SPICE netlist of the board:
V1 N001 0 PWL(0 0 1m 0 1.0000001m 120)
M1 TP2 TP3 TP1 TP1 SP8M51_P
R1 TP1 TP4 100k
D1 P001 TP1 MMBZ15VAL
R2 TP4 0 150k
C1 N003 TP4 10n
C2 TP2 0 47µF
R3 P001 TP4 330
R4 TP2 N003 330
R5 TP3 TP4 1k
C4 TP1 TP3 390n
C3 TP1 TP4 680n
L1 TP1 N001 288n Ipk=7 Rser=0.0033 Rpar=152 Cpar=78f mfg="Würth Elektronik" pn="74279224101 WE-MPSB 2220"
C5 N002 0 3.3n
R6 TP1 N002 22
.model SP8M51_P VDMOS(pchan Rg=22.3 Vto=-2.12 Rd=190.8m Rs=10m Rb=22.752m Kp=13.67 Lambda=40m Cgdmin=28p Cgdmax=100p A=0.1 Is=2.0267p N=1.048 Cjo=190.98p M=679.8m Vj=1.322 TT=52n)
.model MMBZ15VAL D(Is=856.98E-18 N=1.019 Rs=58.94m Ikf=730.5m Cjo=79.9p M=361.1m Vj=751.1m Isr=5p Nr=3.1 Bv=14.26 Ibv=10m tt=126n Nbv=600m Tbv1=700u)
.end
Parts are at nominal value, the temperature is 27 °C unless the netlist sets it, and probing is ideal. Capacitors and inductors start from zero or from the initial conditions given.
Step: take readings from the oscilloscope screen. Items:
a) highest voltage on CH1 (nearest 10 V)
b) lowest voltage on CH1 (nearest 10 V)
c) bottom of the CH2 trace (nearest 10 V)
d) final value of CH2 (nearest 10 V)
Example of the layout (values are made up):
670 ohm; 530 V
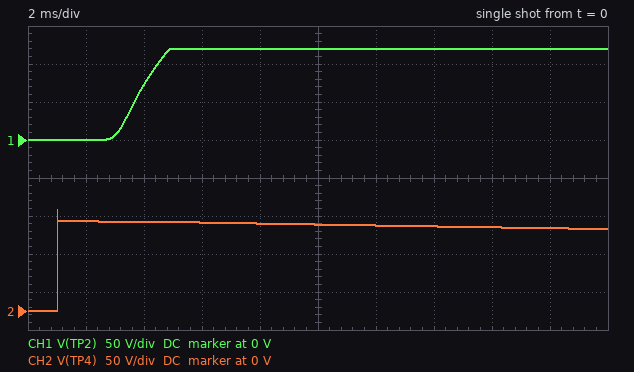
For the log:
120 V; 0 V; 0 V; 110 V
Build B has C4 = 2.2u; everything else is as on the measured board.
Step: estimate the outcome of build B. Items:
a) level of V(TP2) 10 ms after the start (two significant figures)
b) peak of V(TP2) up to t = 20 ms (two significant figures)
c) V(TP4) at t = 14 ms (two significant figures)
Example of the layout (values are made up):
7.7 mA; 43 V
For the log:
73 V; 120 V; 120 V
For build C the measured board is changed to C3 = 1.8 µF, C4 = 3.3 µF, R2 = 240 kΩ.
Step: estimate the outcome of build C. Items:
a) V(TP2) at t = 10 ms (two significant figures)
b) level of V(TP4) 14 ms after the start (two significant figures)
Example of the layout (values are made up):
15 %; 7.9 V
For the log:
25 mV; 120 V
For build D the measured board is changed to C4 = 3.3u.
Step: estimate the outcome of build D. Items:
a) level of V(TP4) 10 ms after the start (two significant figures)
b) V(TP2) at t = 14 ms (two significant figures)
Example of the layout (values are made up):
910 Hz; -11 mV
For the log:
120 V; 95 V
